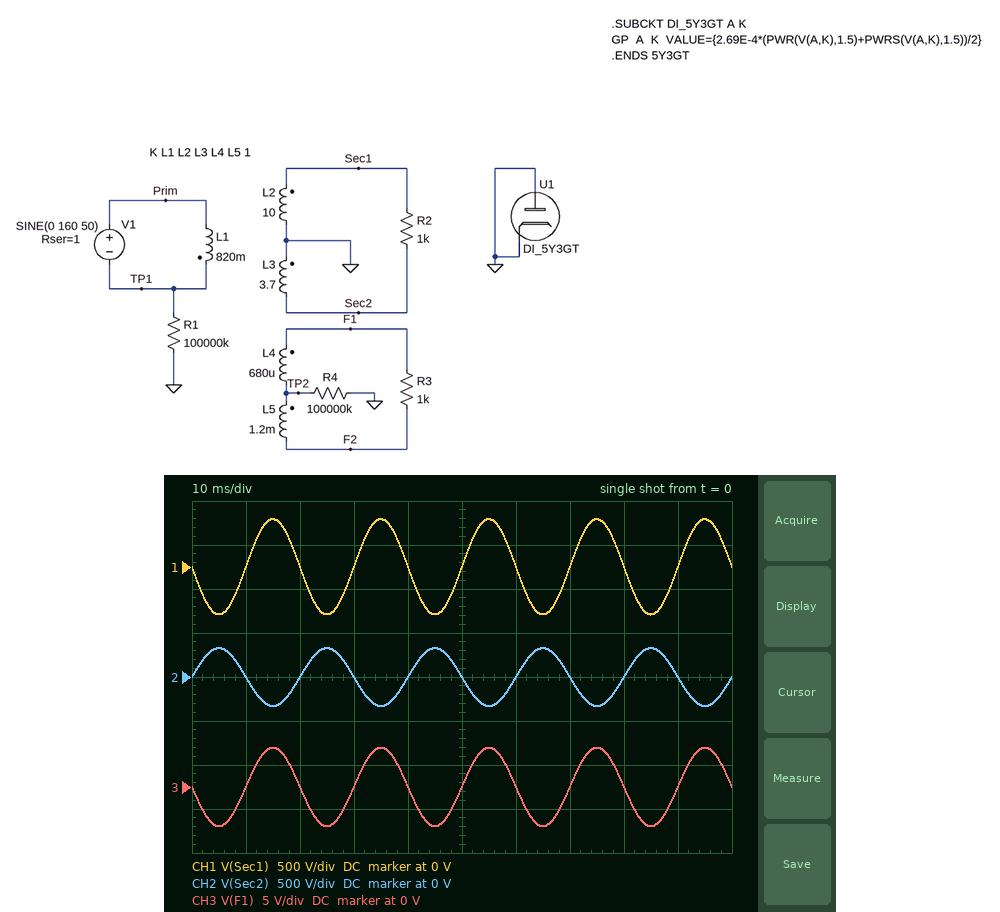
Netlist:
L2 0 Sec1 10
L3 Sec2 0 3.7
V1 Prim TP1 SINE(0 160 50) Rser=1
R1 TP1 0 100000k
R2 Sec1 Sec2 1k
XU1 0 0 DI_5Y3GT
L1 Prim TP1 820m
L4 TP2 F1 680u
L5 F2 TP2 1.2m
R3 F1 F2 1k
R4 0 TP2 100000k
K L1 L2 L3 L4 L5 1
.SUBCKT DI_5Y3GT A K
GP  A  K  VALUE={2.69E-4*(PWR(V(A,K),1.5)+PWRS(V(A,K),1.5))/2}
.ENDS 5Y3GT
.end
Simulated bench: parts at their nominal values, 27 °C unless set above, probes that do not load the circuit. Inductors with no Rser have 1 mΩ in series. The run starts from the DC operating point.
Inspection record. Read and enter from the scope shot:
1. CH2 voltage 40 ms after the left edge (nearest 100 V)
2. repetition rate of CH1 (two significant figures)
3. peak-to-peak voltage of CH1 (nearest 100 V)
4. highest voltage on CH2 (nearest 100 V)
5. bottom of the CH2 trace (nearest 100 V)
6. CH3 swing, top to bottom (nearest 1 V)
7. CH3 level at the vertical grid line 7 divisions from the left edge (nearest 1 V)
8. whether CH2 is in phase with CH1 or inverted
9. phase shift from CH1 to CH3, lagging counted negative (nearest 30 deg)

0 V
50 Hz
1.1 kV
300 V
-300 V
9 V
0 V
inverted
0 deg
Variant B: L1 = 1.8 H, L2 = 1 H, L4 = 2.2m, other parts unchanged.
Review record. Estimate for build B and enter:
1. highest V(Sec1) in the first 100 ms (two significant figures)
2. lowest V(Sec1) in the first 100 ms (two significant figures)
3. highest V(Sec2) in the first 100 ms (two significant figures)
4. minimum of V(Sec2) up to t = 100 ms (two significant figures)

120 V
-120 V
230 V
-230 V
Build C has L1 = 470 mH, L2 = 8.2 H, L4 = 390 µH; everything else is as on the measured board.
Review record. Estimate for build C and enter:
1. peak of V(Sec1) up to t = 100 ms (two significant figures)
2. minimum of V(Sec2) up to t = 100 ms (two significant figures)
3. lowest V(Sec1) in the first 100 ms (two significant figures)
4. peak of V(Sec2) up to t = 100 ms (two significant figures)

640 V
-430 V
-630 V
430 V
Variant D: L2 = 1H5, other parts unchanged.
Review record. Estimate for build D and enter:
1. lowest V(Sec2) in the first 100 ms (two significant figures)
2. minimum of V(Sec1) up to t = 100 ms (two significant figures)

-340 V
-210 V
